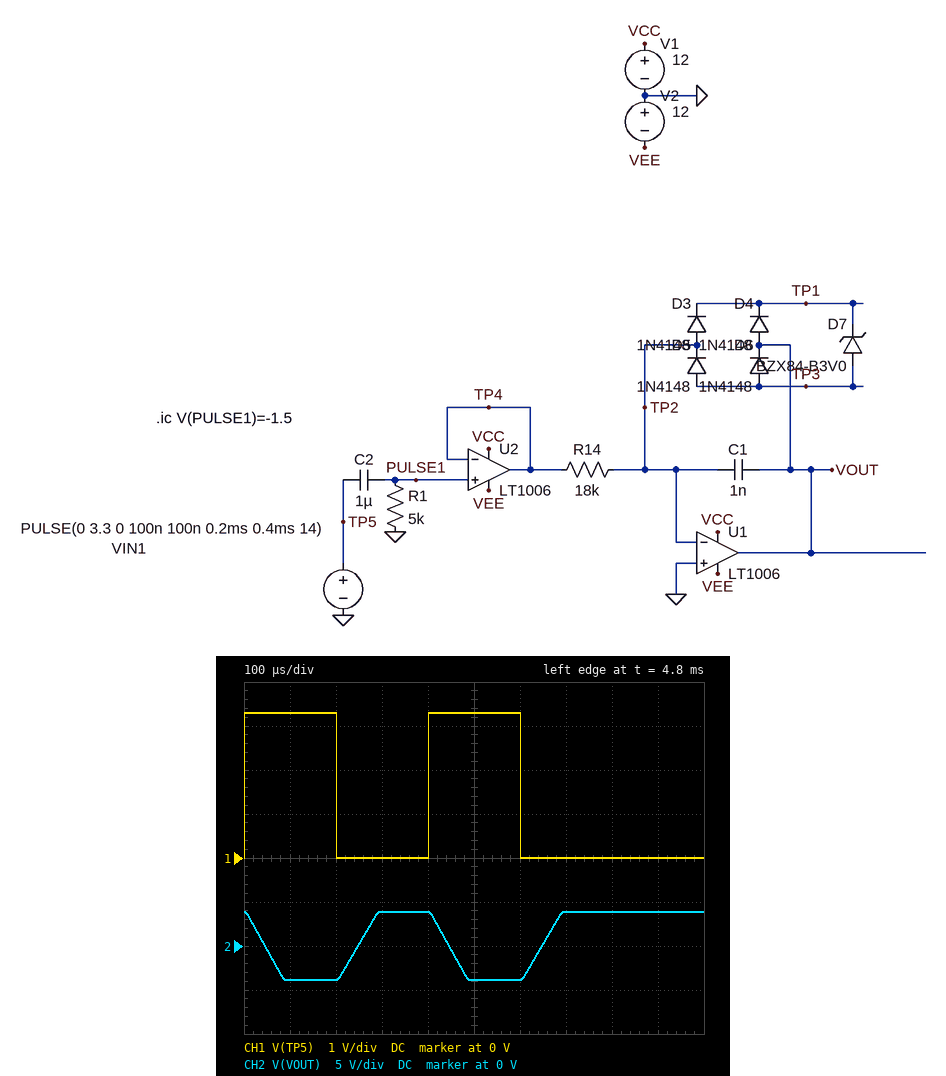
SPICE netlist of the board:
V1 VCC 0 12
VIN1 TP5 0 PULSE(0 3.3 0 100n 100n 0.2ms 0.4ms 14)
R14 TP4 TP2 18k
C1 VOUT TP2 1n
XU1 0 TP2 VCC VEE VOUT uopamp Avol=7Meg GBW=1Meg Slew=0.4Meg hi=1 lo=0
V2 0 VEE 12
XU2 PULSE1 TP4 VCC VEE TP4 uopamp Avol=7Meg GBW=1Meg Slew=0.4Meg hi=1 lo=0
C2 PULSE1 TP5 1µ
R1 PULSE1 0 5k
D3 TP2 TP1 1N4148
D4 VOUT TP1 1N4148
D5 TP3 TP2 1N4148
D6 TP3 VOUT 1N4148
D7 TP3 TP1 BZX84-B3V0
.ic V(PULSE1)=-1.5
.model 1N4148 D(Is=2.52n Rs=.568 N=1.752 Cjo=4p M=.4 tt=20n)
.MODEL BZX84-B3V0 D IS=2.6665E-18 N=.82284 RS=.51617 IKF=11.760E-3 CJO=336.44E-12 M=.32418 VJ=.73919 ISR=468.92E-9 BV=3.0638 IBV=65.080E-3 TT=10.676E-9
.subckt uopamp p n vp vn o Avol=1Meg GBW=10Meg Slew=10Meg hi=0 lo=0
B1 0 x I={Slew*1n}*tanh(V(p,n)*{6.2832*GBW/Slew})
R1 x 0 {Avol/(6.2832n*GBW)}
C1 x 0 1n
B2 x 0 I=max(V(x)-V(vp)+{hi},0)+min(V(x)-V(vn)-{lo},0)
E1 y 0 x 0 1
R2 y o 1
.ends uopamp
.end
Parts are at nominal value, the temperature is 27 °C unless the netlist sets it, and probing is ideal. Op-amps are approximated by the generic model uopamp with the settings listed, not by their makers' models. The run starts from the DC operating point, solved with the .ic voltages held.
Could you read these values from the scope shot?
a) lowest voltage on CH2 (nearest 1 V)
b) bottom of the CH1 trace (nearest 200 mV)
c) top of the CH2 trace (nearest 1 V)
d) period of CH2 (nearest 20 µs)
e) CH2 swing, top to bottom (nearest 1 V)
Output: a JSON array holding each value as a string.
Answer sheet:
["-4 V", "0 V", "4 V", "400 µs", "8 V"]
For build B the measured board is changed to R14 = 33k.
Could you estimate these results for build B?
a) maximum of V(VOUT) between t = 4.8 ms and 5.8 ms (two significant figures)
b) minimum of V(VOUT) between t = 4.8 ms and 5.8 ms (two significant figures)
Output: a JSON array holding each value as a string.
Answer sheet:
["3.8 V", "-3.8 V"]
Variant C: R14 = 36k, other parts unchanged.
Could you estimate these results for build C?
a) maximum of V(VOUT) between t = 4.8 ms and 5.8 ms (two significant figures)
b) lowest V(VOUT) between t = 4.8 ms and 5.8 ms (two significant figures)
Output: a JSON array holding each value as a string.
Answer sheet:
["3.8 V", "-3.8 V"]
